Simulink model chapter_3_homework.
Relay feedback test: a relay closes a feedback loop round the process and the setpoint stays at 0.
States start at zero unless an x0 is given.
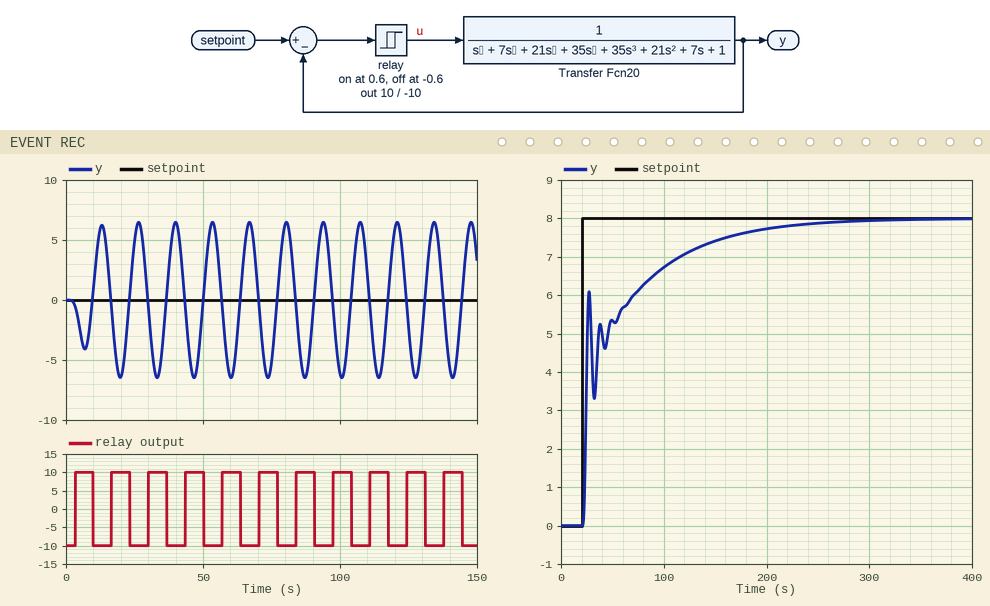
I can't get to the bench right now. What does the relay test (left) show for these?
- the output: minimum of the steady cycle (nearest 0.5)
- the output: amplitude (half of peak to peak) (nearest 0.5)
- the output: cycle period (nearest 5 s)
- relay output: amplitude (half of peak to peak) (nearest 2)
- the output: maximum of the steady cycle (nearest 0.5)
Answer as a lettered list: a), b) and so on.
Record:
a) -6.5
b) 6.5
c) 15 s
d) 10
e) 6.5
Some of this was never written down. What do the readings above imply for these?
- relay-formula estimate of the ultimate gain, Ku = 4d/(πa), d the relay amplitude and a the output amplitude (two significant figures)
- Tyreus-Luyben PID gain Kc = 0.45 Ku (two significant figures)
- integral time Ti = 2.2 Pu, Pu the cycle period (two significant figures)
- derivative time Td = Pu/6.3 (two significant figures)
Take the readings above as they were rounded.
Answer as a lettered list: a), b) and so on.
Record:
a) 2.0
b) 0.90
c) 33 s
d) 2.4 s
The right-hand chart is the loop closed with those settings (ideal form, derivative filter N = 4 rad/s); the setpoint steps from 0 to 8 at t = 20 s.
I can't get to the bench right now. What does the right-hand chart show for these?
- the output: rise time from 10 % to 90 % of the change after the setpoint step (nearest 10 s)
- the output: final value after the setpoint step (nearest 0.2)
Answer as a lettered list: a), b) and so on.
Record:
a) 110 s
b) 8.0
